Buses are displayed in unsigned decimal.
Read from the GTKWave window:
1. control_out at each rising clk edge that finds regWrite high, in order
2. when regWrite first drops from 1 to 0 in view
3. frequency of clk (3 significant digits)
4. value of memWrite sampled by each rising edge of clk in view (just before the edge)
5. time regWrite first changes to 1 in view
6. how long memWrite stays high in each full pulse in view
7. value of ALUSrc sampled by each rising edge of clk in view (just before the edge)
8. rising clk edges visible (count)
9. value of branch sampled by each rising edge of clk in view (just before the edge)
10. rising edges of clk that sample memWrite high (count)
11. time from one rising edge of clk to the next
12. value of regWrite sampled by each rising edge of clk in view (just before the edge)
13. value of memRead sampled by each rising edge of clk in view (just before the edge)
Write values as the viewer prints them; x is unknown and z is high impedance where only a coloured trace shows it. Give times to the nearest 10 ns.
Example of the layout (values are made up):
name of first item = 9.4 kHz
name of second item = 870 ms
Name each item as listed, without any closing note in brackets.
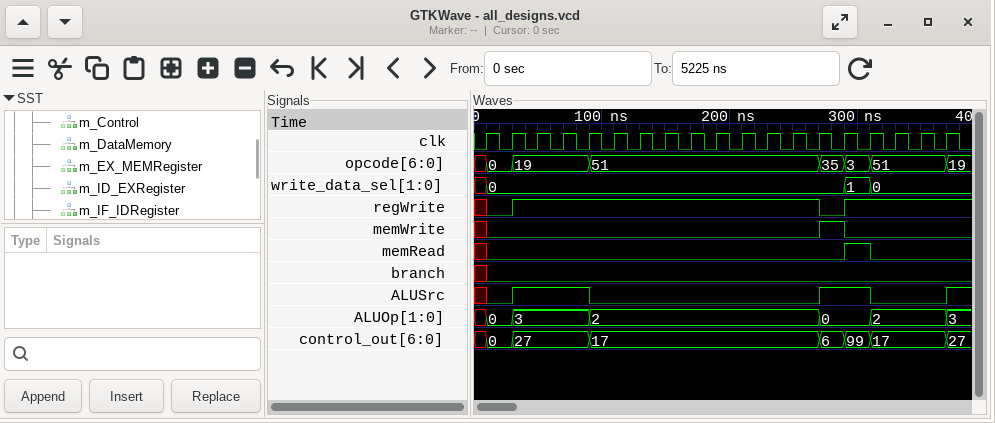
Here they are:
control_out at each rising clk edge that finds regWrite high, in order = 27, 27, 27, 17, 17, 17, 17, 17, 17, 17, 17, 17, 99, 17, 17, 17
when regWrite first drops from 1 to 0 in view = 270 ns
frequency of clk = 50.0 MHz
value of memWrite sampled by each rising edge of clk in view = x 0 0 0 0 0 0 0 0 0 0 0 0 0 1 0 0 0 0
time regWrite first changes to 1 in view = 30 ns
how long memWrite stays high in each full pulse in view = 20 ns
value of ALUSrc sampled by each rising edge of clk in view = x 0 1 1 1 0 0 0 0 0 0 0 0 0 1 1 0 0 0
rising clk edges visible = 19
value of branch sampled by each rising edge of clk in view = x 0 0 0 0 0 0 0 0 0 0 0 0 0 0 0 0 0 0
rising edges of clk that sample memWrite high = 1
time from one rising edge of clk to the next = 20 ns
value of regWrite sampled by each rising edge of clk in view = x 0 1 1 1 1 1 1 1 1 1 1 1 1 0 1 1 1 1
value of memRead sampled by each rising edge of clk in view = x 0 0 0 0 0 0 0 0 0 0 0 0 0 0 1 0 0 0
